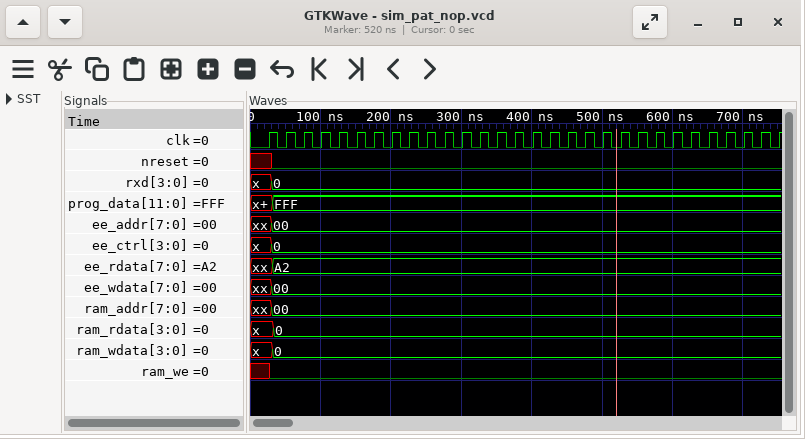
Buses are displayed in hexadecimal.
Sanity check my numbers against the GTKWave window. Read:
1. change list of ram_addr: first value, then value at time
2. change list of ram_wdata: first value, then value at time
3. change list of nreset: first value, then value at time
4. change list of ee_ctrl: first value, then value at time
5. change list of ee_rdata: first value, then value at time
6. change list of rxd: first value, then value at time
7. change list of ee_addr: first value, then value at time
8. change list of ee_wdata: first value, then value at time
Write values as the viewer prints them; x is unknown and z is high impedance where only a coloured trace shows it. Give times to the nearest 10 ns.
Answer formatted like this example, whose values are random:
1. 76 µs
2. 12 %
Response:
1. xx, 00 at 30 ns
2. x, 0 at 30 ns
3. x, 0 at 30 ns
4. x, 0 at 30 ns
5. xx, A2 at 30 ns
6. x, 0 at 30 ns
7. xx, 00 at 30 ns
8. xx, 00 at 30 ns
